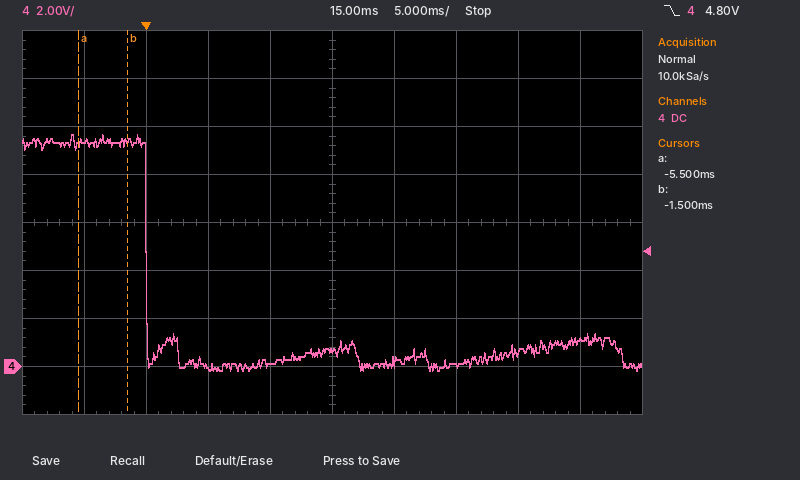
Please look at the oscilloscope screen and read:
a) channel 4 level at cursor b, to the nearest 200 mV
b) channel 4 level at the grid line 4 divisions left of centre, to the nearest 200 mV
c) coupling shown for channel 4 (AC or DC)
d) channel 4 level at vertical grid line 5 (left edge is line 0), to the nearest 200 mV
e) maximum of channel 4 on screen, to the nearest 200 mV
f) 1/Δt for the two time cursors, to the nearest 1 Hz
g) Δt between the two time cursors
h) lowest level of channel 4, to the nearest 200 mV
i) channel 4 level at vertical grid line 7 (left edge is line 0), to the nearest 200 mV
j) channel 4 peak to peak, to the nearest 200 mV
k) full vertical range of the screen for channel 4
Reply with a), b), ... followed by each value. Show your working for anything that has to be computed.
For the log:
a) 9.4 V
b) 9.4 V
c) DC
d) 600 mV
e) 9.6 V
f) 1 / 4.0 ms ≈ 250 Hz
g) -1.5 ms − (-5.5 ms) = 4.0 ms
h) -200 mV
i) 0.0 V
j) 9.6 V − (-200 mV) = 9.8 V
k) 16 V
